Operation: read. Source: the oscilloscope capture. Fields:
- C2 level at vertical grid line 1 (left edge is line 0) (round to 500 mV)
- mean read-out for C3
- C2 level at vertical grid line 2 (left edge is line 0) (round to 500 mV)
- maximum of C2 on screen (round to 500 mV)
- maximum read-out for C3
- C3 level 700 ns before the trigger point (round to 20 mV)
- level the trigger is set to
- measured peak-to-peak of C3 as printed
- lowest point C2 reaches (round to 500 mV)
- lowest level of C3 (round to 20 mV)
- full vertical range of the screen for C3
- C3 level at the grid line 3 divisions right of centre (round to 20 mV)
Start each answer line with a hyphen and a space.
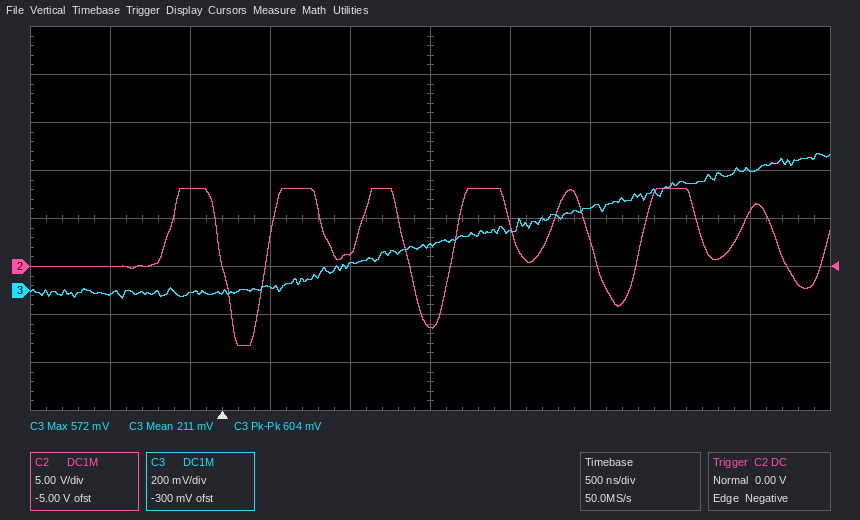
- 0.0 V
- 211 mV
- 8.0 V
- 8.0 V
- 572 mV
- -20 mV
- 0.00 V
- 604 mV
- -8.0 V
- -40 mV
- 1.6 V
- 440 mV
